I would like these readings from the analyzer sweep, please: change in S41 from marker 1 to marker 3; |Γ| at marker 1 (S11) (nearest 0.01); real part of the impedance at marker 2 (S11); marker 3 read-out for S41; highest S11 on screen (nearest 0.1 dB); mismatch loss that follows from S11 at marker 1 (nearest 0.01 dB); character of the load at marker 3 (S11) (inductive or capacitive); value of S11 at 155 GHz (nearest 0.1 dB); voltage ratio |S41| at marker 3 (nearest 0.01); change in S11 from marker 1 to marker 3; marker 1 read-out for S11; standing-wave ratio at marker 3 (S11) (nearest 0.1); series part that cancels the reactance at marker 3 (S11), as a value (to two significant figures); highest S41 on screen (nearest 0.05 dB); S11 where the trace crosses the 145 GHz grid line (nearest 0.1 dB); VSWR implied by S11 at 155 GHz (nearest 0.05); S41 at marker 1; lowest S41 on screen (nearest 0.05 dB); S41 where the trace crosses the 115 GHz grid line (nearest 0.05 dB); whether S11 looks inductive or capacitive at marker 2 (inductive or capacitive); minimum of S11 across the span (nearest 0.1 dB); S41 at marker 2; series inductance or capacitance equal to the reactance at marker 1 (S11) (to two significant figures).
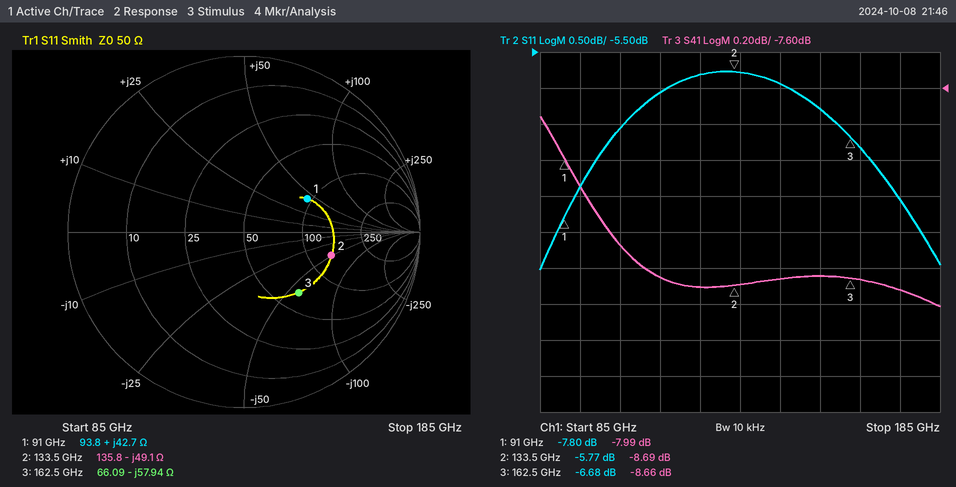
-0.67 dB
0.41
135.8 Ω
-8.66 dB
-5.8 dB
0.79 dB
capacitive
-6.3 dB
0.37
1.12 dB
-7.80 dB
2.7
57 pH
-7.75 dB
-5.9 dB
2.90
-7.99 dB
-8.80 dB
-8.65 dB
capacitive
-8.5 dB
-8.69 dB
75 pH
